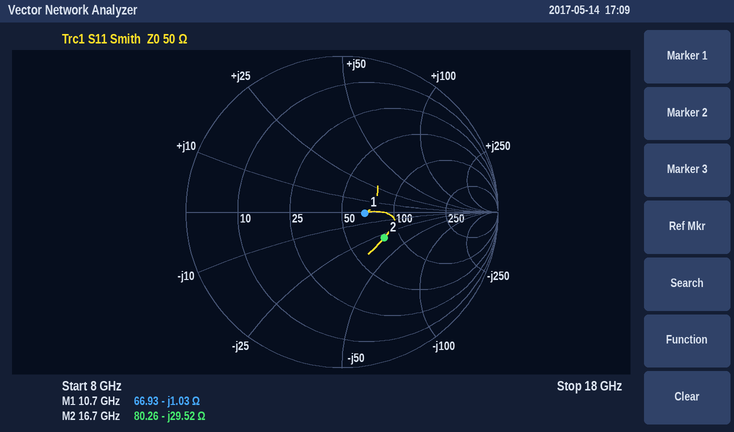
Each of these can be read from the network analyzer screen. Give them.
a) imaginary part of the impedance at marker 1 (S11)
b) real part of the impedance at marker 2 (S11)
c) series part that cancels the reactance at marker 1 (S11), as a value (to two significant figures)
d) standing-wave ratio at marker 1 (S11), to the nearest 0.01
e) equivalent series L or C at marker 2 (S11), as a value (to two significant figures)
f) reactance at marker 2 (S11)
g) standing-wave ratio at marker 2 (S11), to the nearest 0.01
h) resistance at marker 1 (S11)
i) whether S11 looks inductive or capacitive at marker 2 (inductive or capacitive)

-1.03 Ω
80.26 Ω
15 pH
1.34
320 fF
-29.52 Ω
1.93
66.93 Ω
capacitive
